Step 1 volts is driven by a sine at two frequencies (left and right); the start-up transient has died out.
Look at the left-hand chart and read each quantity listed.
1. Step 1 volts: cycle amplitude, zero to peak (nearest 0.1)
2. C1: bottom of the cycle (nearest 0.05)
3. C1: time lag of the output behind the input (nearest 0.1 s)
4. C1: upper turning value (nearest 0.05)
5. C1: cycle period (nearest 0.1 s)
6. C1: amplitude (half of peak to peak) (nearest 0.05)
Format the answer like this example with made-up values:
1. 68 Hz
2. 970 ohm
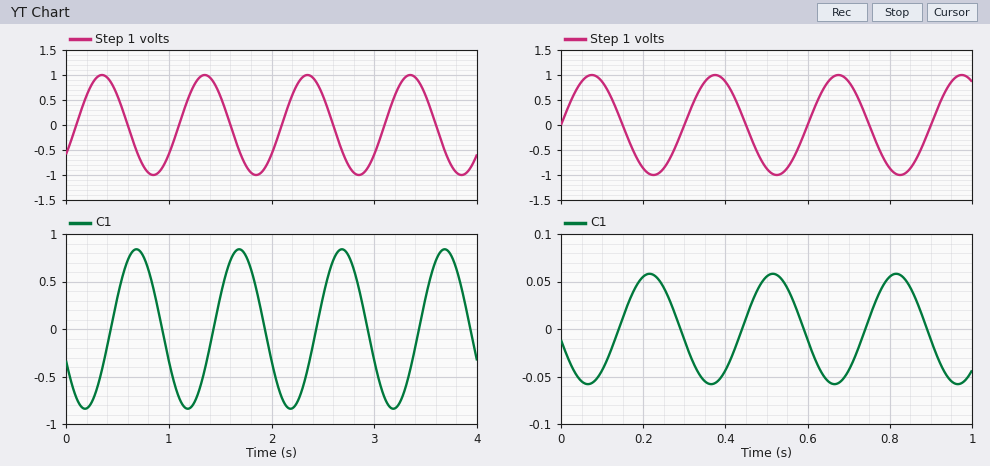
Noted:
1. 1.0
2. -0.85
3. 0.3 s
4. 0.85
5. 1.0 s
6. 0.85
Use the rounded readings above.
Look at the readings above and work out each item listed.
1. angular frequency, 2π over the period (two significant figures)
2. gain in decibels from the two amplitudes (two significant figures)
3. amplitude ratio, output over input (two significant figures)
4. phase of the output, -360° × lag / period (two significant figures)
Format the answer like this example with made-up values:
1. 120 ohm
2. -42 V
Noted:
1. 6.3 rad/s
2. -1.4 dB
3. 0.85
4. -110°
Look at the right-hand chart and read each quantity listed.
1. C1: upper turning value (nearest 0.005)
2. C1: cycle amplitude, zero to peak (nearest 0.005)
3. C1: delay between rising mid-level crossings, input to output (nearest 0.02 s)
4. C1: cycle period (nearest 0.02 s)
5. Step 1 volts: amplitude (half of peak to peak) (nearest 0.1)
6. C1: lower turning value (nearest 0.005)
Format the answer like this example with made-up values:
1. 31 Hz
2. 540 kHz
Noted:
1. 0.060
2. 0.060
3. 0.14 s
4. 0.30 s
5. 1.0
6. -0.060
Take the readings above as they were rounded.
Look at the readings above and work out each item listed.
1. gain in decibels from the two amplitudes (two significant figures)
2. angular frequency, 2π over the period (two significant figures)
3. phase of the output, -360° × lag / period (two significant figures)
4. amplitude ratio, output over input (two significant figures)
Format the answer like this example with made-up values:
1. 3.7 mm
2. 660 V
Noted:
1. -24 dB
2. 21 rad/s
3. -170°
4. 0.060
